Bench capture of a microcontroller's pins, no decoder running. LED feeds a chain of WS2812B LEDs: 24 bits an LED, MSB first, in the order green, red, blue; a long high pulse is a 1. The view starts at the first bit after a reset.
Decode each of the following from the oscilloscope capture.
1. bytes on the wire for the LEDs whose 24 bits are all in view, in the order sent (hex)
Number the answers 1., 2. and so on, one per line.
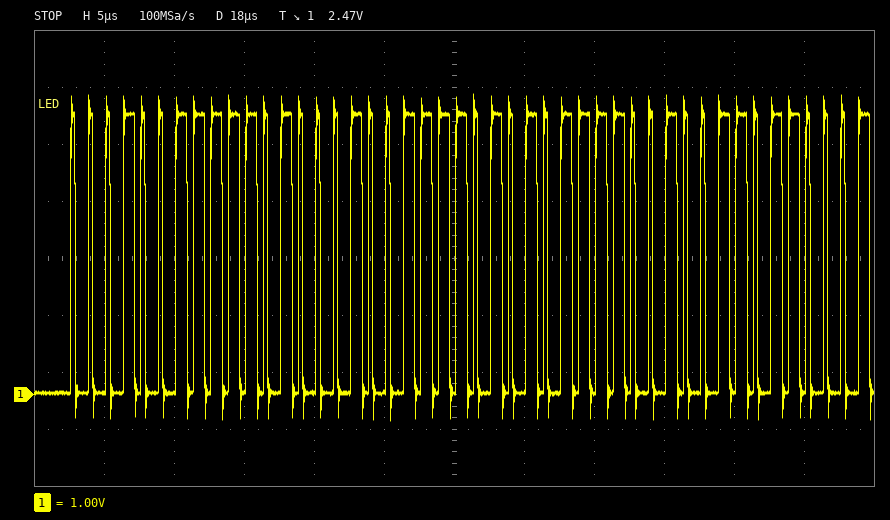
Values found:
1. 13 E8 9E
